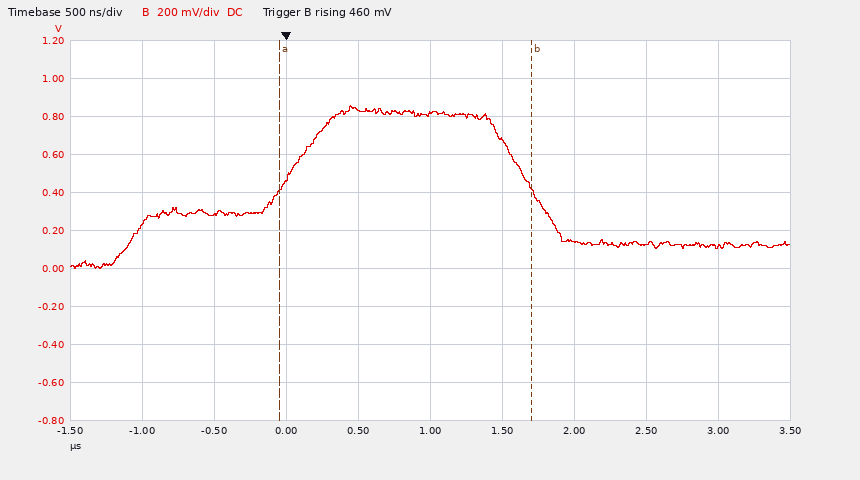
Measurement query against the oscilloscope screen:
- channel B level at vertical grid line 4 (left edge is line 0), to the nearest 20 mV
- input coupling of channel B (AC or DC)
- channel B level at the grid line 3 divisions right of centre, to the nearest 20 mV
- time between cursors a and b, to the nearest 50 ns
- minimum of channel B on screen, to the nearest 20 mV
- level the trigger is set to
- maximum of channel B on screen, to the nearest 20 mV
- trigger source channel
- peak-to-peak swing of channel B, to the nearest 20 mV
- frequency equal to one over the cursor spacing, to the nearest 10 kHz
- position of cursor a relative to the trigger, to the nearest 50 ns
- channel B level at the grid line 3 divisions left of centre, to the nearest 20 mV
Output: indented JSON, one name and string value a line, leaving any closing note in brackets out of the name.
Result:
{
  "channel B level at vertical grid line 4 (left edge is line 0), to the nearest 20 mV": "840 mV",
  "input coupling of channel B": "DC",
  "channel B level at the grid line 3 divisions right of centre, to the nearest 20 mV": "120 mV",
  "time between cursors a and b, to the nearest 50 ns": "1.75 µs",
  "minimum of channel B on screen, to the nearest 20 mV": "0 mV",
  "level the trigger is set to": "460 mV",
  "maximum of channel B on screen, to the nearest 20 mV": "860 mV",
  "trigger source channel": "channel B",
  "peak-to-peak swing of channel B, to the nearest 20 mV": "860 mV",
  "frequency equal to one over the cursor spacing, to the nearest 10 kHz": "570 kHz",
  "position of cursor a relative to the trigger, to the nearest 50 ns": "-50 ns",
  "channel B level at the grid line 3 divisions left of centre, to the nearest 20 mV": "280 mV"
}
